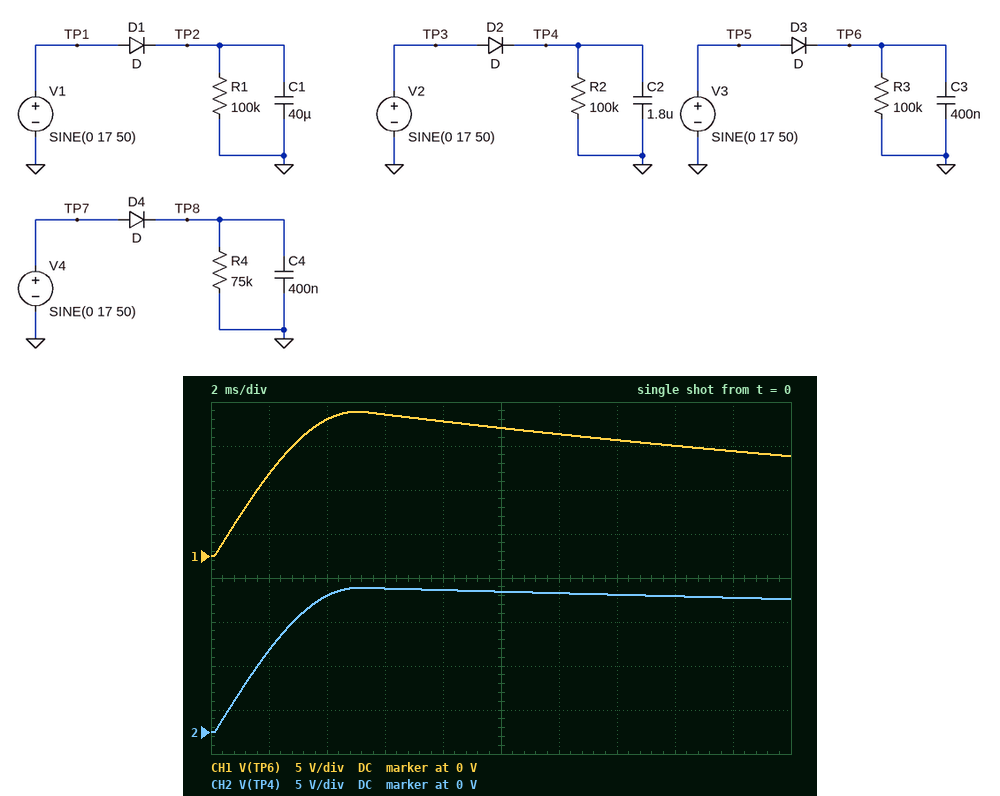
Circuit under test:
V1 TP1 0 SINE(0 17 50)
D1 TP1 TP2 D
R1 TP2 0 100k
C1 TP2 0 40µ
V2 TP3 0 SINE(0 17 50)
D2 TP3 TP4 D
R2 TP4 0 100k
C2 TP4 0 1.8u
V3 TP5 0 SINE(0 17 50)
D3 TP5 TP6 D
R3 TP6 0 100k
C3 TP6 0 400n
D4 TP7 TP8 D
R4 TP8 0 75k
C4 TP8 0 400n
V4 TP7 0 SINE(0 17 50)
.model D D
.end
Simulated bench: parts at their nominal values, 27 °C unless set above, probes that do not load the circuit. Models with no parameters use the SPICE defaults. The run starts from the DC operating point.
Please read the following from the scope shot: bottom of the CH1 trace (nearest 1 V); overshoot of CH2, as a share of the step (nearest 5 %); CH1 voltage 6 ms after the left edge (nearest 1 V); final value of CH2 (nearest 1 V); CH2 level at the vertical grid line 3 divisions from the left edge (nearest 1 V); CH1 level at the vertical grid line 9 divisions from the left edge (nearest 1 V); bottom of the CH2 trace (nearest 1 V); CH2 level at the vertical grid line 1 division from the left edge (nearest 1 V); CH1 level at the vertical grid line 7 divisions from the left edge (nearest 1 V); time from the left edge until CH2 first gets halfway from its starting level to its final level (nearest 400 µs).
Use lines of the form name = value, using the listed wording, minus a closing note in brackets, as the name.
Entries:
bottom of the CH1 trace = 0 V
overshoot of CH2, as a share of the step = 10 %
CH1 voltage 6 ms after the left edge = 16 V
final value of CH2 = 15 V
CH2 level at the vertical grid line 3 divisions from the left edge = 16 V
CH1 level at the vertical grid line 9 divisions from the left edge = 12 V
bottom of the CH2 trace = 0 V
CH2 level at the vertical grid line 1 division from the left edge = 9 V
CH1 level at the vertical grid line 7 divisions from the left edge = 13 V
time from the left edge until CH2 first gets halfway from its starting level to its final level = 1.6 ms
